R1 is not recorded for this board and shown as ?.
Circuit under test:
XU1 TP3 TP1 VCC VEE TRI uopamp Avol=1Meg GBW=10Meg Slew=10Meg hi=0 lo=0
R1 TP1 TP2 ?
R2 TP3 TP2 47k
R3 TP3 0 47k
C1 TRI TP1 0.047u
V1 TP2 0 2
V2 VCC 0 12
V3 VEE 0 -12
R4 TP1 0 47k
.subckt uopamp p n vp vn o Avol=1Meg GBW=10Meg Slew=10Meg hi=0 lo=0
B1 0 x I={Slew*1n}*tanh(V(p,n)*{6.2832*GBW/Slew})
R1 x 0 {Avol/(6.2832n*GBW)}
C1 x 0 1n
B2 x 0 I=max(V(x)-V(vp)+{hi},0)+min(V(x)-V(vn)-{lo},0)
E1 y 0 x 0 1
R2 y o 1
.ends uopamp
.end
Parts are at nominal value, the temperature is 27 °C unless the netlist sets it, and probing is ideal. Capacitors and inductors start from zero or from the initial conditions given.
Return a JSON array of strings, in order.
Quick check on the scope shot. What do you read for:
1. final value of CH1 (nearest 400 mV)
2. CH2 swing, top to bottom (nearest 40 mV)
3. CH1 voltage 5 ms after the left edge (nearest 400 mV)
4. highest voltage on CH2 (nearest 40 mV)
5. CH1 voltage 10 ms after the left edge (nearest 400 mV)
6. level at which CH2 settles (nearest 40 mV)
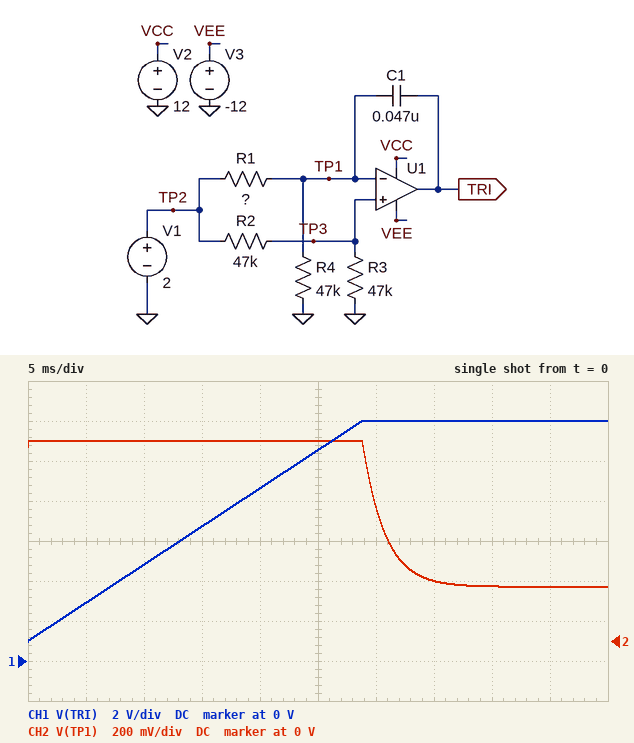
["12.0 V", "720 mV", "2.8 V", "1.00 V", "4.8 V", "280 mV"]
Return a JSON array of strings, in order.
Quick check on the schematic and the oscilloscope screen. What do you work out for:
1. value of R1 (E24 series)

["300 kΩ"]
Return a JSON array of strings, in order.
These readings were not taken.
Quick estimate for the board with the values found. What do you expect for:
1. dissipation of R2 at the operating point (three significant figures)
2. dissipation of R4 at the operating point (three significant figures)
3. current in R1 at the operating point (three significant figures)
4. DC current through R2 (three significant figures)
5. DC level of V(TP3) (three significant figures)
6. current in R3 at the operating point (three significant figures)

["21.3 µW", "1.56 µW", "5.76 µA", "21.3 µA", "1.00 V", "21.3 µA"]
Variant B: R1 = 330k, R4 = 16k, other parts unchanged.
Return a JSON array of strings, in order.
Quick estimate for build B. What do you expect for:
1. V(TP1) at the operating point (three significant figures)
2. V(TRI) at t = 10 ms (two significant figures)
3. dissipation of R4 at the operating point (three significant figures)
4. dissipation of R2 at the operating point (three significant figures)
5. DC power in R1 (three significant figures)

["92.5 mV", "12 V", "535 nW", "21.3 µW", "11.0 µW"]
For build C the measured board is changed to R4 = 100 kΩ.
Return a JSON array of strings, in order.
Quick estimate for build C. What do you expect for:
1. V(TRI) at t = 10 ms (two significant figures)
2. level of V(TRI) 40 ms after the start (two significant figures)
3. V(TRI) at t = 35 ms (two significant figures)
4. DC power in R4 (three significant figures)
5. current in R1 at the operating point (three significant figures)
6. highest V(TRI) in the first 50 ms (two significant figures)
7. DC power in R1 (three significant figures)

["2.4 V", "6.7 V", "6.0 V", "2.50 µW", "5.00 µA", "8.1 V", "7.50 µW"]
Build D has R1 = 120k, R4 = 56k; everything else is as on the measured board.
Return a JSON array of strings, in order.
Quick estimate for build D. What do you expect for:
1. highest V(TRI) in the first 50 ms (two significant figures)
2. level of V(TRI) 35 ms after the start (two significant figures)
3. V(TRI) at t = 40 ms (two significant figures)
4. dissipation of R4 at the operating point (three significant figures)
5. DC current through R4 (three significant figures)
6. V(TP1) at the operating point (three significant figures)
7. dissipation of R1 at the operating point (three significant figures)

["11 V", "8.1 V", "9.1 V", "7.23 µW", "11.4 µA", "636 mV", "15.5 µW"]
